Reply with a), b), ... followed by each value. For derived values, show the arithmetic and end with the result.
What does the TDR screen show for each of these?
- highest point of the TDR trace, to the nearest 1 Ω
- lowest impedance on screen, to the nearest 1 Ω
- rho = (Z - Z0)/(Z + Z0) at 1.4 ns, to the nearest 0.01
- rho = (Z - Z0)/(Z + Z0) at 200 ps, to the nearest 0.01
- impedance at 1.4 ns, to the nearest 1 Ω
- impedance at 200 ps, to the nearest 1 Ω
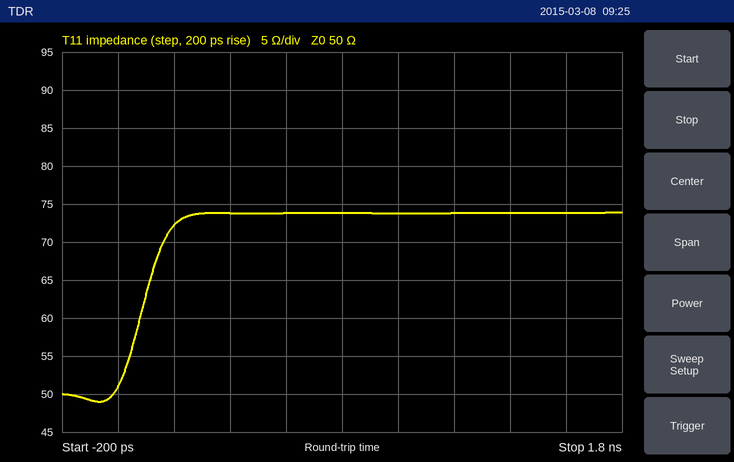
a) 74 Ω
b) 49 Ω
c) (74 − 50)/(74 + 50) ≈ +0.19
d) (72 − 50)/(72 + 50) ≈ +0.18
e) 74 Ω
f) 72 Ω
